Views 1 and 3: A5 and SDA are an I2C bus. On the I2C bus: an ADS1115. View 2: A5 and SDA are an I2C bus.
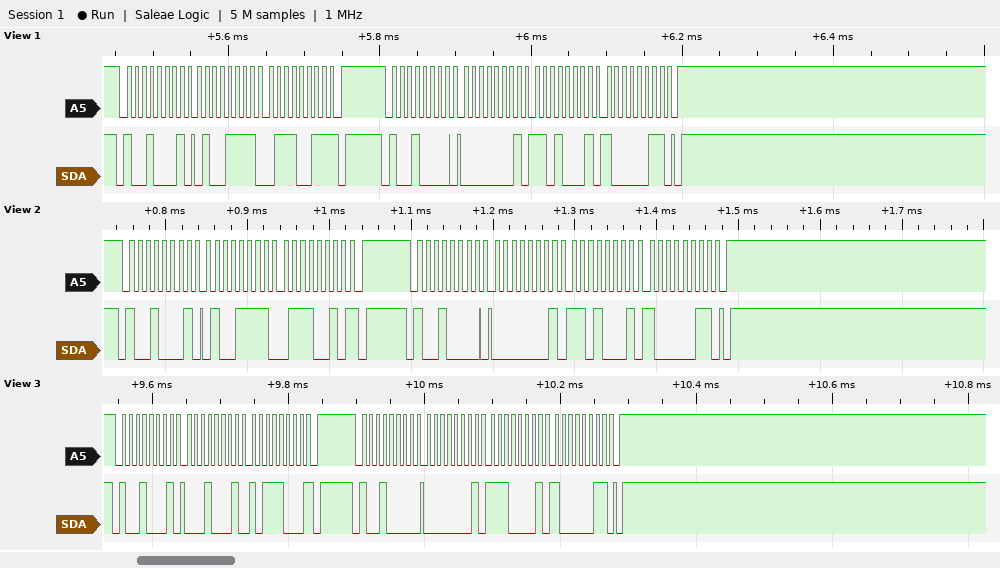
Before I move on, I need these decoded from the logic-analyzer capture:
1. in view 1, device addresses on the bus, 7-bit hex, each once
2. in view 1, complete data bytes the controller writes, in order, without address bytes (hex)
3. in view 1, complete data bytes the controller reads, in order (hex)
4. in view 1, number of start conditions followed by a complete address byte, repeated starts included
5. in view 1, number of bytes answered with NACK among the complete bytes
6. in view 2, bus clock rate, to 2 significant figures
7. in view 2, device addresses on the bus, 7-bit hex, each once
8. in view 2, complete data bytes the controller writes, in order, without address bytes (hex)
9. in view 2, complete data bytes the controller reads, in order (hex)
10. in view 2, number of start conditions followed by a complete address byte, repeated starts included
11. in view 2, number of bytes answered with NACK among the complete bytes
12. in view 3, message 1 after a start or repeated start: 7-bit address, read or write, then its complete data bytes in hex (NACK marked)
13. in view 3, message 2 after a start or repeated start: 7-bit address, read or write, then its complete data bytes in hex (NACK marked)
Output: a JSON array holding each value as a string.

["0x48", "01 D1 83", "4F 73", "2", "1", "100 kHz", "0x48", "01 D1 83", "4F 72", "2", "1", "0x48 read: 11 B8 NACK", "0x48 write: 01 E1 83"]
